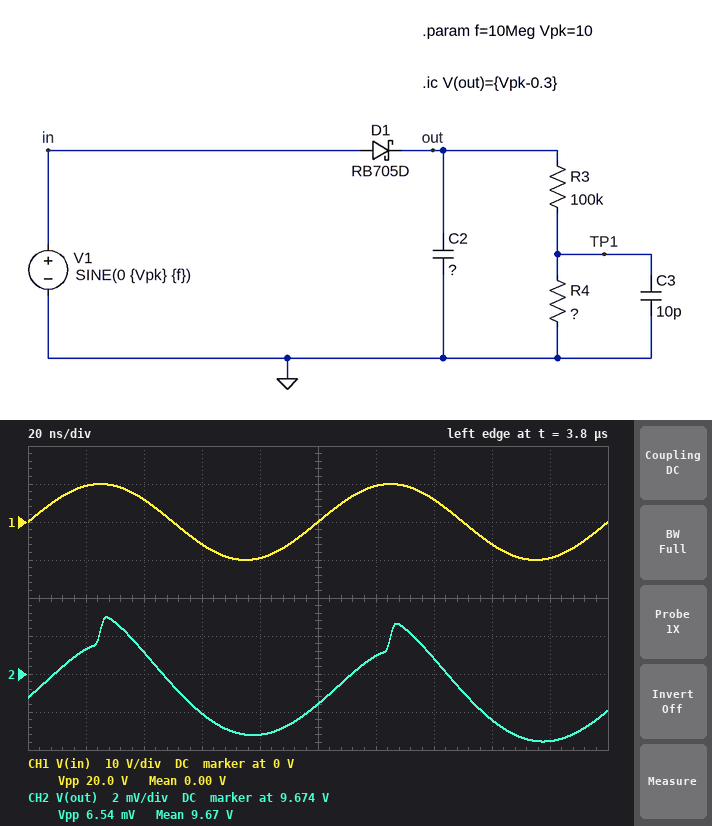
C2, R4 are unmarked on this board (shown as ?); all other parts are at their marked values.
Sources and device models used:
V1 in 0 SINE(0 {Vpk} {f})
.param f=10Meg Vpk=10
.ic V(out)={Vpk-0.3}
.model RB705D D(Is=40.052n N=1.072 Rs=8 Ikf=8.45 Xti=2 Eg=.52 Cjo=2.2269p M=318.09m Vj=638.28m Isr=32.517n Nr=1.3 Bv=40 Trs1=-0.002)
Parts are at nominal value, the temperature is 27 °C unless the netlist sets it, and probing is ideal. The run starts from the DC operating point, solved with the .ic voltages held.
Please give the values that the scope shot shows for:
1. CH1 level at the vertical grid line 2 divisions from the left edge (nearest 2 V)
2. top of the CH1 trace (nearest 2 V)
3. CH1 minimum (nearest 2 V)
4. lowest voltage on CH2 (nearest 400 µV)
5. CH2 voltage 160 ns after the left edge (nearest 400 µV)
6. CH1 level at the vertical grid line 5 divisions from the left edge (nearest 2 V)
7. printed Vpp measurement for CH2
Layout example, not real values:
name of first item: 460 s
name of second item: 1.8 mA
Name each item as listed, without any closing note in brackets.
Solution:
CH1 level at the vertical grid line 2 divisions from the left edge: 6 V
top of the CH1 trace: 10 V
CH1 minimum: -10 V
lowest voltage on CH2: 9.6704 V
CH2 voltage 160 ns after the left edge: 9.6716 V
CH1 level at the vertical grid line 5 divisions from the left edge: 0 V
printed Vpp measurement for CH2: 6.54 mV
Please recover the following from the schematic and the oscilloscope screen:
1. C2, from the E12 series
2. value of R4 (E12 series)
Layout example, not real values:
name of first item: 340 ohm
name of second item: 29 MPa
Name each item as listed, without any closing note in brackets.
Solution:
C2, from the E12 series: 3.9 nF
value of R4: 27 kΩ
